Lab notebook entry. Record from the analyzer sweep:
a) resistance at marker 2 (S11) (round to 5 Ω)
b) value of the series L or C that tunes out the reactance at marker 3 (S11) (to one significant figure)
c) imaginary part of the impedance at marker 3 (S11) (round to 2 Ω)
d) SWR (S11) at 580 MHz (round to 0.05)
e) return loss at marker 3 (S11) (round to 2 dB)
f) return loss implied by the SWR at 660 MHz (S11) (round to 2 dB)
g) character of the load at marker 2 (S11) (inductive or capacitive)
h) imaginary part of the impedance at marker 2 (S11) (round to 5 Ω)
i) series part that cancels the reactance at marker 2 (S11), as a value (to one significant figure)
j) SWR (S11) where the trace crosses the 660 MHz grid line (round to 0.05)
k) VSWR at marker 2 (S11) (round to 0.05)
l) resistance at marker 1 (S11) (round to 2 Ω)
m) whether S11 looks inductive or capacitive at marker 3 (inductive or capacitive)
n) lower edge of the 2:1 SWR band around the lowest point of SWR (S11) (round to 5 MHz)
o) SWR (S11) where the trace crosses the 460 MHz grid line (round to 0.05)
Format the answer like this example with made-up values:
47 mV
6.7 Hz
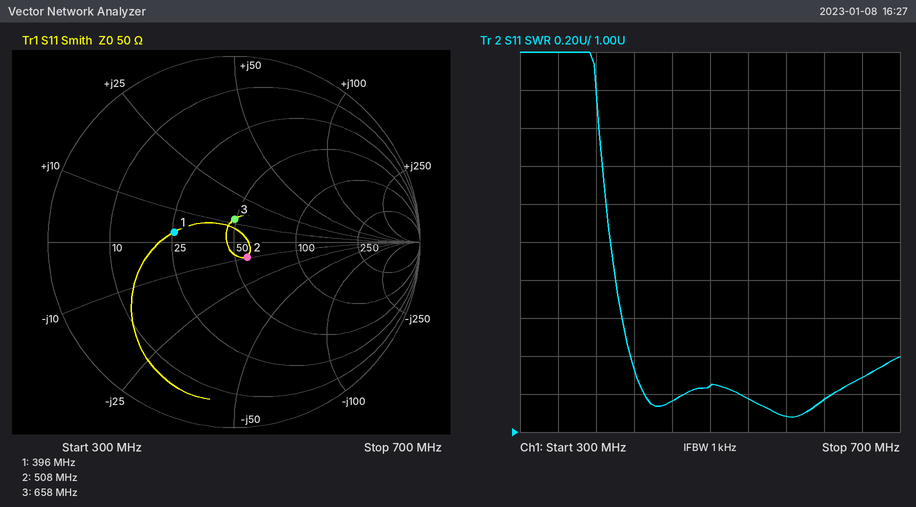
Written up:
55 Ω
20 pF
+12 Ω
1.10
18 dB
18 dB
capacitive
-10 Ω
3 nH
1.30
1.25
26 Ω
inductive
395 MHz
1.15
